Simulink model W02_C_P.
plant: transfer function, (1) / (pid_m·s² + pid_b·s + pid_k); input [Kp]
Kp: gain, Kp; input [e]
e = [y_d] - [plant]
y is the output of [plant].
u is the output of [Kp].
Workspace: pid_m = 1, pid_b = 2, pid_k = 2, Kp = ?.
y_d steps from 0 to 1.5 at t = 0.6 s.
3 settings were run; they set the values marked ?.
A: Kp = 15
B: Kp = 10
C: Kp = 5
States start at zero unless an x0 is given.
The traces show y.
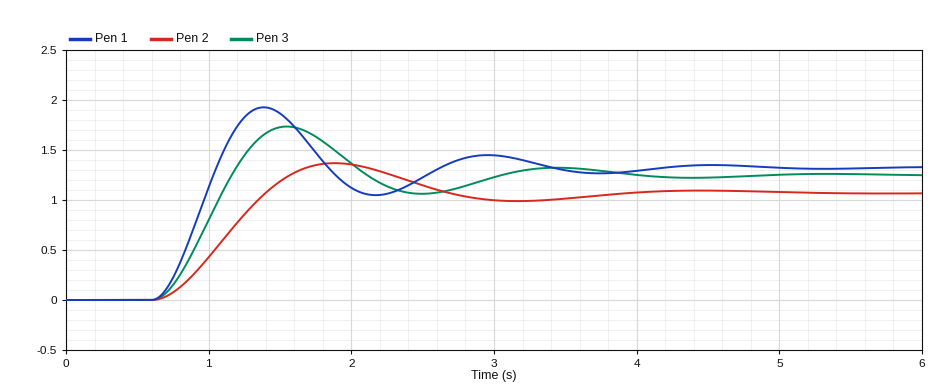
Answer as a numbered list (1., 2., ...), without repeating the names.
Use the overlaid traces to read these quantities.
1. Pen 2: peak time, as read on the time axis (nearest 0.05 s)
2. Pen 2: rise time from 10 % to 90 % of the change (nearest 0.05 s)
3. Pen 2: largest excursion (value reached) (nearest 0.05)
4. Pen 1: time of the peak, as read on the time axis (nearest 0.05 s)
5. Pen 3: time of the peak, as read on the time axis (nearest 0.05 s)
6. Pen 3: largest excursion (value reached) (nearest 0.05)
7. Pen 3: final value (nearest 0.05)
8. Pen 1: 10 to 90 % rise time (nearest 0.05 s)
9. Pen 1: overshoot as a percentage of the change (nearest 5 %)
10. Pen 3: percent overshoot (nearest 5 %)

1. 1.90 s
2. 0.55 s
3. 1.35
4. 1.40 s
5. 1.55 s
6. 1.75
7. 1.25
8. 0.30 s
9. 45 %
10. 40 %
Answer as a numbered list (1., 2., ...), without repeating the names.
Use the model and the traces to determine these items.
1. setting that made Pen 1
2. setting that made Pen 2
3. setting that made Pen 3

1. A
2. C
3. B
